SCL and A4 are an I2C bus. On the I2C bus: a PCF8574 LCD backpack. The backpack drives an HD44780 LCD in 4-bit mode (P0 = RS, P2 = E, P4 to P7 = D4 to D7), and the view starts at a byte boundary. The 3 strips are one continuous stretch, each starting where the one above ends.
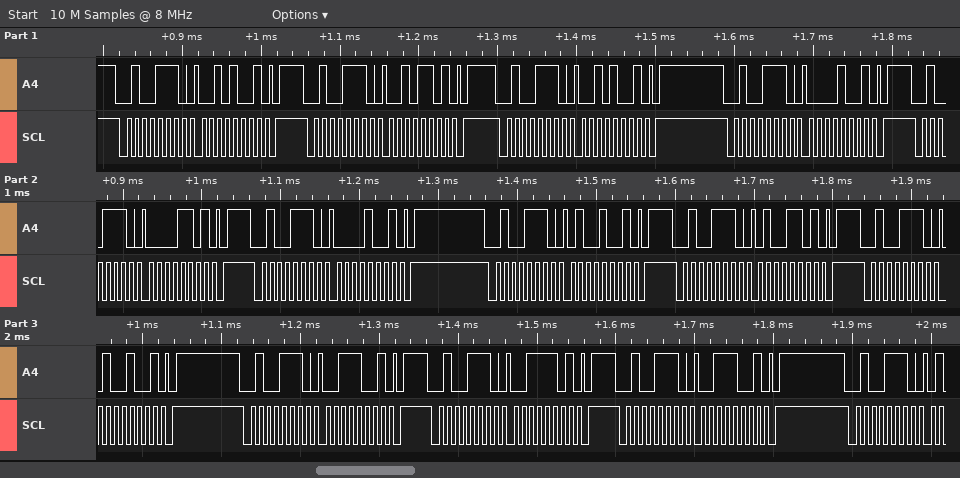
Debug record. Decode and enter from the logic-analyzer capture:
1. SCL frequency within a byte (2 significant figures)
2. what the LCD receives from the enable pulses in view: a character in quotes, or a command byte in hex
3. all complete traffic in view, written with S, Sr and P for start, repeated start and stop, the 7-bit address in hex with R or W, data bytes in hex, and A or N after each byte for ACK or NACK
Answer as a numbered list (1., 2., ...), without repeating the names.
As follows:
1. 100 kHz
2. ' ' 'C'
3. S 27W A 29 A P S 27W A 2D A P S 27W A 29 A P S 27W A 09 A P S 27W A 0D A P S 27W A 09 A P S 27W A 49 A P S 27W A 4D A P S 27W A 49 A P S 27W A 39 A P S 27W A 3D A P S 27W A 39 A P S 27W A
